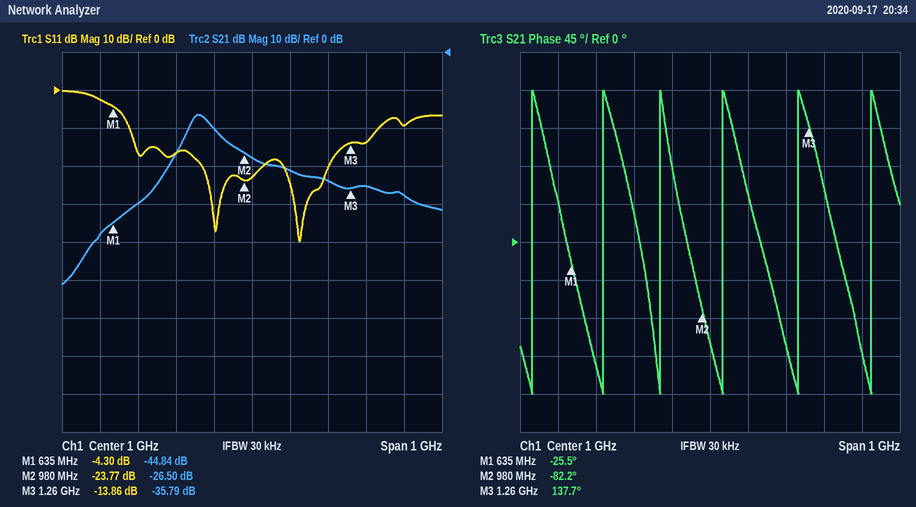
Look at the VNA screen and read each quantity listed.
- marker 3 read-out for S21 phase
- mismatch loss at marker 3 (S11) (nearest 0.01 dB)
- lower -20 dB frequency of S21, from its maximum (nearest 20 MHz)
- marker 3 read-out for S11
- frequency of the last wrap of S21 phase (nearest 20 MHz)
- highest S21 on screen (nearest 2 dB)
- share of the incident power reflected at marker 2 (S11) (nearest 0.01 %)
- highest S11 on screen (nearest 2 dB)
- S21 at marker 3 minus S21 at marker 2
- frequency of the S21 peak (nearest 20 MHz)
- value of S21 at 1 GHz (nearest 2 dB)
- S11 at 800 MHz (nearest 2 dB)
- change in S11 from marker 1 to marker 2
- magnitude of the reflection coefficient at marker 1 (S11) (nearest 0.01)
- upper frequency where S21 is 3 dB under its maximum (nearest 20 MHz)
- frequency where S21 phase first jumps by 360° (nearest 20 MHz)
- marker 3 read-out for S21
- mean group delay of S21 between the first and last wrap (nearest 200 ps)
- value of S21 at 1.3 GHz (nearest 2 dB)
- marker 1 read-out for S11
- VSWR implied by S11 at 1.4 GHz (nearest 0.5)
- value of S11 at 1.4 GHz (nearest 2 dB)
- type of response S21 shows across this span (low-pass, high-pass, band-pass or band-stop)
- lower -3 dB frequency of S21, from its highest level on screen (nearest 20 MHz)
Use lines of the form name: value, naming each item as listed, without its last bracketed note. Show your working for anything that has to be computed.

marker 3 read-out for S21 phase: 137.7°
mismatch loss at marker 3 (S11): −10 log10(1 − 10^(-13.86/10)) ≈ 0.18 dB
lower -20 dB frequency of S21, from its maximum: 740 MHz
marker 3 read-out for S11: -13.86 dB
frequency of the last wrap of S21 phase: 1.42 GHz
highest S21 on screen: -16 dB
share of the incident power reflected at marker 2 (S11): 10^(-23.77/10) ≈ 0.42 %
highest S11 on screen: 0 dB
S21 at marker 3 minus S21 at marker 2: -35.79 − (-26.5) = -9.29 dB
frequency of the S21 peak: 860 MHz
value of S21 at 1 GHz: -28 dB
S11 at 800 MHz: -16 dB
change in S11 from marker 1 to marker 2: -23.77 − (-4.3) = -19.47 dB
magnitude of the reflection coefficient at marker 1 (S11): 10^(-4.3/20) ≈ 0.61
upper frequency where S21 is 3 dB under its maximum: 900 MHz
frequency where S21 phase first jumps by 360°: 540 MHz
marker 3 read-out for S21: -35.79 dB
mean group delay of S21 between the first and last wrap: 5 cycles / (1.42 GHz − 540 MHz) ≈ 5.68 ns, so 5.6 ns to the nearest 200 ps
value of S21 at 1.3 GHz: -36 dB
marker 1 read-out for S11: -4.30 dB
VSWR implied by S11 at 1.4 GHz: |Γ| = 10^(-10/20) = 0.3162; VSWR = (1 + 0.3162)/(1 − 0.3162) ≈ 1.92, so 2.0 to the nearest 0.5
value of S11 at 1.4 GHz: -10 dB
type of response S21 shows across this span: band-pass
lower -3 dB frequency of S21, from its highest level on screen: 840 MHz
